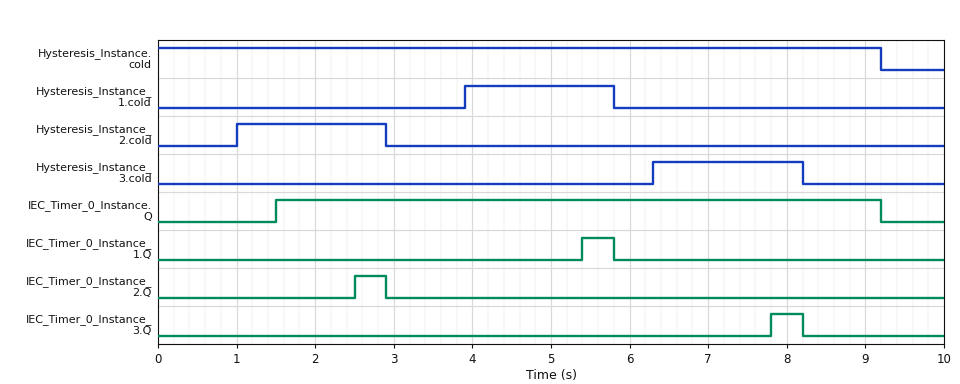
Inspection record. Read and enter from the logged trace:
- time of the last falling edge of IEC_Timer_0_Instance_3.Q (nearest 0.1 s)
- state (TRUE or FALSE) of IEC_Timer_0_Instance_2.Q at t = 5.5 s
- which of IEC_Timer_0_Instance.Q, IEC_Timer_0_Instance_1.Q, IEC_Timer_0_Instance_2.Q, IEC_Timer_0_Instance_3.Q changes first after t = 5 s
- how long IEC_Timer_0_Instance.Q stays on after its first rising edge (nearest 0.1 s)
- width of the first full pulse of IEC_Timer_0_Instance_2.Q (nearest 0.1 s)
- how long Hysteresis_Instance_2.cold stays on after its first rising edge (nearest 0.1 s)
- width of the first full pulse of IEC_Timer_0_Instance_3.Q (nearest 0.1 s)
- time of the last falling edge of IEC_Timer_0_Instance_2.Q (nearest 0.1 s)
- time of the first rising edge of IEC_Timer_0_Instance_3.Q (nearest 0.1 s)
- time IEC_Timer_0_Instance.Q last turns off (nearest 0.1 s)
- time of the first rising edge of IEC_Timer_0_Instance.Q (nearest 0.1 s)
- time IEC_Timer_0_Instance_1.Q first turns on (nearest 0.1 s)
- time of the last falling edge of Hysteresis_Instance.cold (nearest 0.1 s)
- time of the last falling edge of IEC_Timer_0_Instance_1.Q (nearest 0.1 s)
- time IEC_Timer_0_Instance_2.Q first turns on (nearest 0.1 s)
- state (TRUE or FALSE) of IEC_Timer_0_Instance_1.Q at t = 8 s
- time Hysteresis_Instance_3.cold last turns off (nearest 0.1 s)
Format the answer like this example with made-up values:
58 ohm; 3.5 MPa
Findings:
8.2 s; FALSE; IEC_Timer_0_Instance_1.Q; 7.7 s; 0.4 s; 1.9 s; 0.4 s; 2.9 s; 7.8 s; 9.2 s; 1.5 s; 5.4 s; 9.2 s; 5.8 s; 2.5 s; FALSE; 8.2 s
